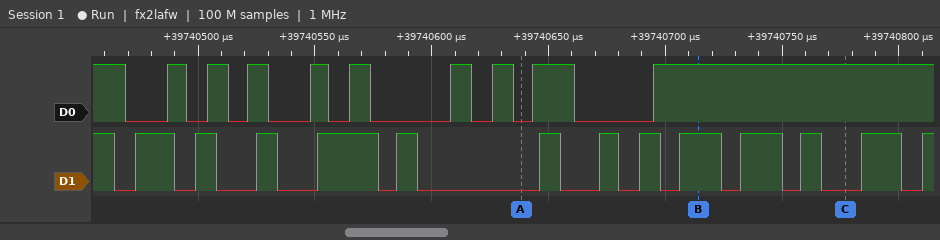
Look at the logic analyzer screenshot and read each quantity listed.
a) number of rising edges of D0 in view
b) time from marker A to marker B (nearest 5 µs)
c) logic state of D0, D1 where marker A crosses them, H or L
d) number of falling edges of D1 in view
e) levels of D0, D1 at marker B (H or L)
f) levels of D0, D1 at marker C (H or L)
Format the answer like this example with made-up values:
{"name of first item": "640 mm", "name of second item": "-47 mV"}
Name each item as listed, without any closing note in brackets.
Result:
{"number of rising edges of D0 in view": "9", "time from marker A to marker B": "75 µs", "logic state of D0, D1 where marker A crosses them, H or L": "D0=L, D1=L", "number of falling edges of D1 in view": "13", "levels of D0, D1 at marker B": "D0=H, D1=H", "levels of D0, D1 at marker C": "D0=H, D1=L"}
